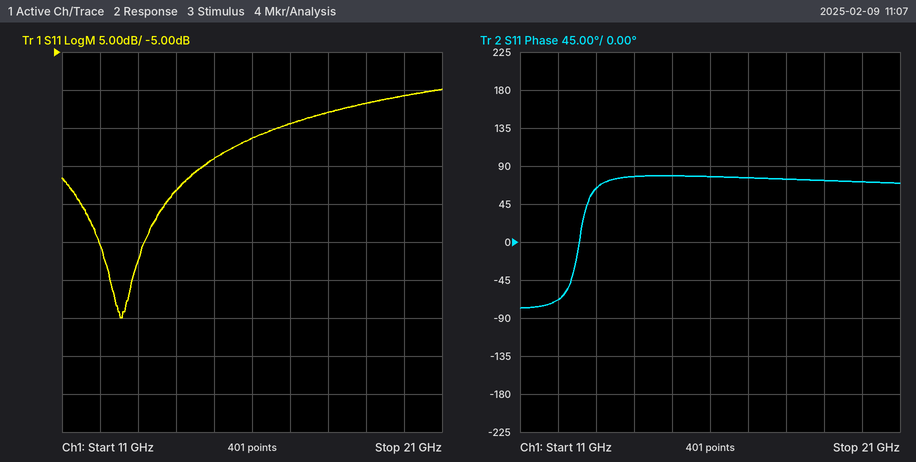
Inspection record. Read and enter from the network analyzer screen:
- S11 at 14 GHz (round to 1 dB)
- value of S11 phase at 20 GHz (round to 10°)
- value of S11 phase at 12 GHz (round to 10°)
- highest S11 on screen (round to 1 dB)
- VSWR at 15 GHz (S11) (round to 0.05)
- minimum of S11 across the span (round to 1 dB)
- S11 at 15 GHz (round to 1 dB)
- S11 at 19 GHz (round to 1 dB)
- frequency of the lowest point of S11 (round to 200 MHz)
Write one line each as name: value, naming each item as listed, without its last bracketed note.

S11 at 14 GHz: -23 dB
value of S11 phase at 20 GHz: 70°
value of S11 phase at 12 GHz: -70°
highest S11 on screen: -10 dB
VSWR at 15 GHz (S11): 1.25
minimum of S11 across the span: -40 dB
S11 at 15 GHz: -19 dB
S11 at 19 GHz: -12 dB
frequency of the lowest point of S11: 12.6 GHz
